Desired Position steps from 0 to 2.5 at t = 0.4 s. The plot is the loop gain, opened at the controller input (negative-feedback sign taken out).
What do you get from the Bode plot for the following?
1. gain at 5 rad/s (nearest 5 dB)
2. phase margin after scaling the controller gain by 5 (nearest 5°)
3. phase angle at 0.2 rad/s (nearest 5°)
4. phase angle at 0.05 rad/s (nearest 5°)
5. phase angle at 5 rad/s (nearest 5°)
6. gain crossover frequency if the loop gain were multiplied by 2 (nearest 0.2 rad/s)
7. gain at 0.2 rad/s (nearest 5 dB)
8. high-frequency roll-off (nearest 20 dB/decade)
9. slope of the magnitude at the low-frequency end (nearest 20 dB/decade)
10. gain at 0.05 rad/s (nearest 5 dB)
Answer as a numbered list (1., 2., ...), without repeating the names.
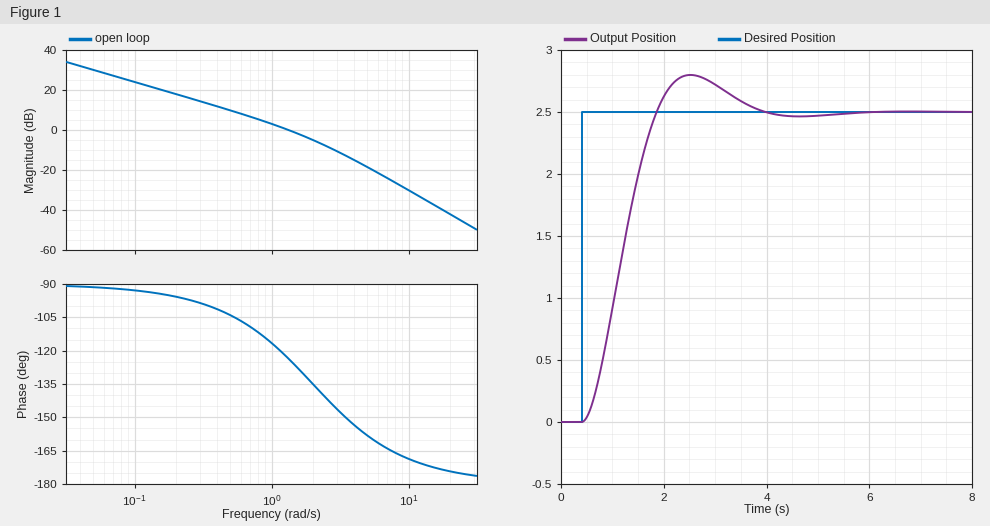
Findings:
1. -20 dB
2. 30°
3. -95°
4. -90°
5. -160°
6. 2.2 rad/s
7. 20 dB
8. -40 dB/decade
9. -20 dB/decade
10. 30 dB
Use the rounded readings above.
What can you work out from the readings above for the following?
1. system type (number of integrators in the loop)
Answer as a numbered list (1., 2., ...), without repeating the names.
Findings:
1. 1
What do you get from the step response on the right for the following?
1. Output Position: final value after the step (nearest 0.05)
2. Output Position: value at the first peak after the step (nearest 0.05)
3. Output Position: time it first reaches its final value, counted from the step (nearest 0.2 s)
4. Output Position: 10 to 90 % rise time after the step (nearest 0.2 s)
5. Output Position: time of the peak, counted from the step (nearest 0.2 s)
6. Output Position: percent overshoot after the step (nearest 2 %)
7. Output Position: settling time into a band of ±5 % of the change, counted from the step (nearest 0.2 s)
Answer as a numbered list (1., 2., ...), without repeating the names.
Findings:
1. 2.50
2. 2.80
3. 1.4 s
4. 1.0 s
5. 2.2 s
6. 12 %
7. 3.0 s
